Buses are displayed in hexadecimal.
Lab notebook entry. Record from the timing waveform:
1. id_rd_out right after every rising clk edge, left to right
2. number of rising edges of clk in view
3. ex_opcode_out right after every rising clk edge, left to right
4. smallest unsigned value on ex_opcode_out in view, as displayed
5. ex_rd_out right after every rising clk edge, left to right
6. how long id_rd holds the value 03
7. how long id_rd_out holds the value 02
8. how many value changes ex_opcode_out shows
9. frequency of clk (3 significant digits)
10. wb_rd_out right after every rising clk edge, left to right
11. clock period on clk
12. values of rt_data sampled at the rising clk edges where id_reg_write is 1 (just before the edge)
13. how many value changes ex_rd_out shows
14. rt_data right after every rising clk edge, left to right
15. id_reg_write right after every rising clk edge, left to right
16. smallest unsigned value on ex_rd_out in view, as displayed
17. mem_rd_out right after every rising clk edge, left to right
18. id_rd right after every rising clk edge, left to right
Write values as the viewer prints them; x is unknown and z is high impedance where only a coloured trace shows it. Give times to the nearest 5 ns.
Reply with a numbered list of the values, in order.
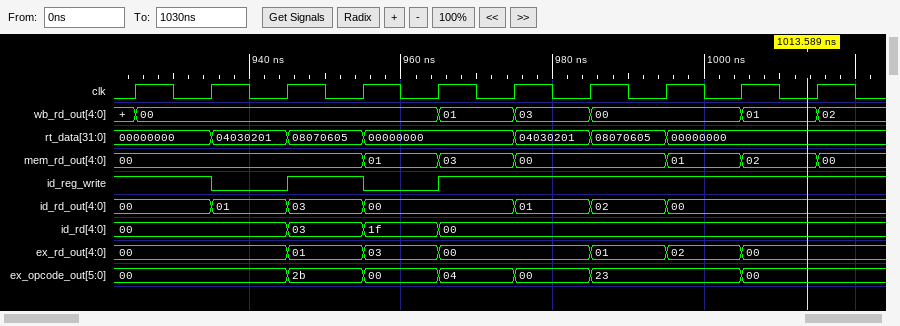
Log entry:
1. 00, 01, 03, 00, 00, 01, 02, 00, 00, 00
2. 10
3. 00, 00, 2b, 00, 04, 00, 23, 23, 00, 00
4. 00
5. 00, 00, 01, 03, 00, 00, 01, 02, 00, 00
6. 10 ns
7. 10 ns
8. 6
9. 100 MHz
10. 00, 00, 00, 00, 01, 03, 00, 00, 01, 02
11. 10 ns
12. 00000000, 00000000, 08070605, 00000000, 04030201, 08070605, 00000000, 00000000
13. 6
14. 00000000, 04030201, 08070605, 00000000, 00000000, 04030201, 08070605, 00000000, 00000000, 00000000
15. 1 0 1 0 1 1 1 1 1 1
16. 00
17. 00, 00, 00, 01, 03, 00, 00, 01, 02, 00
18. 00, 00, 03, 1f, 00, 00, 00, 00, 00, 00
